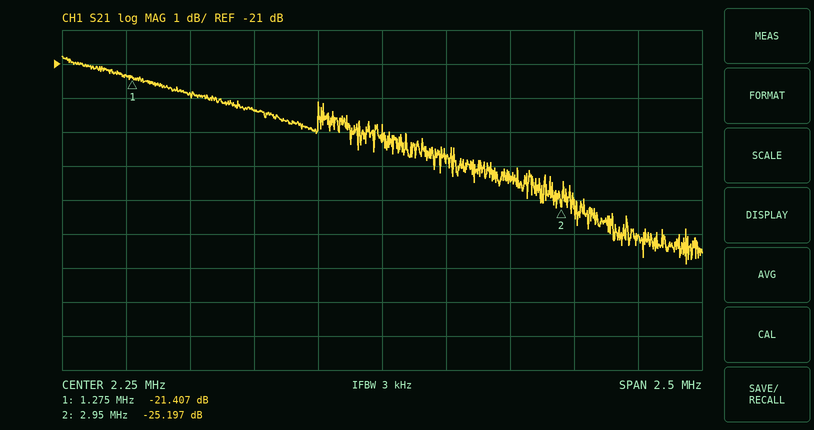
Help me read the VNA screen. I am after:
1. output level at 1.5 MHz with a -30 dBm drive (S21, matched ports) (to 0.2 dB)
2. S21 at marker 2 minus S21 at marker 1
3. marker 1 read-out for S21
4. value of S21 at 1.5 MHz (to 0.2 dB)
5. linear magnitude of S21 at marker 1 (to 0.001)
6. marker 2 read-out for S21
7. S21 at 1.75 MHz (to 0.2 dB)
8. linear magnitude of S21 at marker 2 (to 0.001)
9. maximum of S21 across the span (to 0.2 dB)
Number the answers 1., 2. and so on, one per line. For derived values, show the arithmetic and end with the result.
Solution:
1. -30 dBm + (-21.8 dB) = -51.8 dBm
2. -25.197 − (-21.407) = -3.790 dB
3. -21.407 dB
4. -21.8 dB
5. 10^(-21.407/20) ≈ 0.085
6. -25.197 dB
7. -22.4 dB
8. 10^(-25.197/20) ≈ 0.055
9. -20.8 dB
